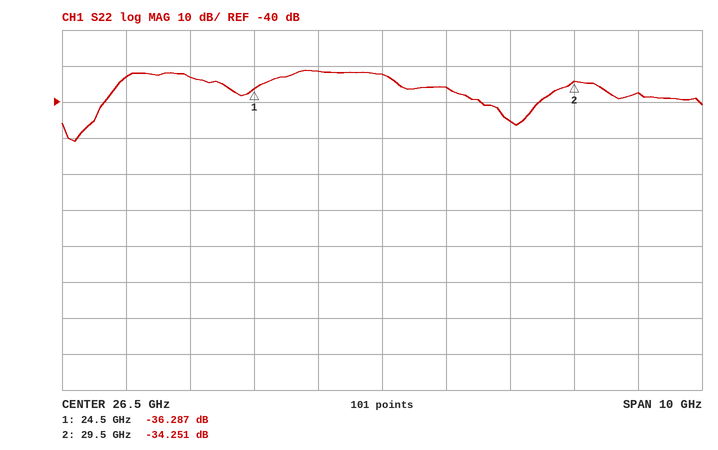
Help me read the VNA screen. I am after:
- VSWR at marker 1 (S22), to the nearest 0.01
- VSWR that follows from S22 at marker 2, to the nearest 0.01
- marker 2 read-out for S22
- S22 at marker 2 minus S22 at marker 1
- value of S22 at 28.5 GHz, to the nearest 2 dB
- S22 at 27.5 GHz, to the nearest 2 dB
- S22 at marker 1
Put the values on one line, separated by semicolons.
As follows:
1.03; 1.04; -34.251 dB; 2.036 dB; -46 dB; -36 dB; -36.287 dB
